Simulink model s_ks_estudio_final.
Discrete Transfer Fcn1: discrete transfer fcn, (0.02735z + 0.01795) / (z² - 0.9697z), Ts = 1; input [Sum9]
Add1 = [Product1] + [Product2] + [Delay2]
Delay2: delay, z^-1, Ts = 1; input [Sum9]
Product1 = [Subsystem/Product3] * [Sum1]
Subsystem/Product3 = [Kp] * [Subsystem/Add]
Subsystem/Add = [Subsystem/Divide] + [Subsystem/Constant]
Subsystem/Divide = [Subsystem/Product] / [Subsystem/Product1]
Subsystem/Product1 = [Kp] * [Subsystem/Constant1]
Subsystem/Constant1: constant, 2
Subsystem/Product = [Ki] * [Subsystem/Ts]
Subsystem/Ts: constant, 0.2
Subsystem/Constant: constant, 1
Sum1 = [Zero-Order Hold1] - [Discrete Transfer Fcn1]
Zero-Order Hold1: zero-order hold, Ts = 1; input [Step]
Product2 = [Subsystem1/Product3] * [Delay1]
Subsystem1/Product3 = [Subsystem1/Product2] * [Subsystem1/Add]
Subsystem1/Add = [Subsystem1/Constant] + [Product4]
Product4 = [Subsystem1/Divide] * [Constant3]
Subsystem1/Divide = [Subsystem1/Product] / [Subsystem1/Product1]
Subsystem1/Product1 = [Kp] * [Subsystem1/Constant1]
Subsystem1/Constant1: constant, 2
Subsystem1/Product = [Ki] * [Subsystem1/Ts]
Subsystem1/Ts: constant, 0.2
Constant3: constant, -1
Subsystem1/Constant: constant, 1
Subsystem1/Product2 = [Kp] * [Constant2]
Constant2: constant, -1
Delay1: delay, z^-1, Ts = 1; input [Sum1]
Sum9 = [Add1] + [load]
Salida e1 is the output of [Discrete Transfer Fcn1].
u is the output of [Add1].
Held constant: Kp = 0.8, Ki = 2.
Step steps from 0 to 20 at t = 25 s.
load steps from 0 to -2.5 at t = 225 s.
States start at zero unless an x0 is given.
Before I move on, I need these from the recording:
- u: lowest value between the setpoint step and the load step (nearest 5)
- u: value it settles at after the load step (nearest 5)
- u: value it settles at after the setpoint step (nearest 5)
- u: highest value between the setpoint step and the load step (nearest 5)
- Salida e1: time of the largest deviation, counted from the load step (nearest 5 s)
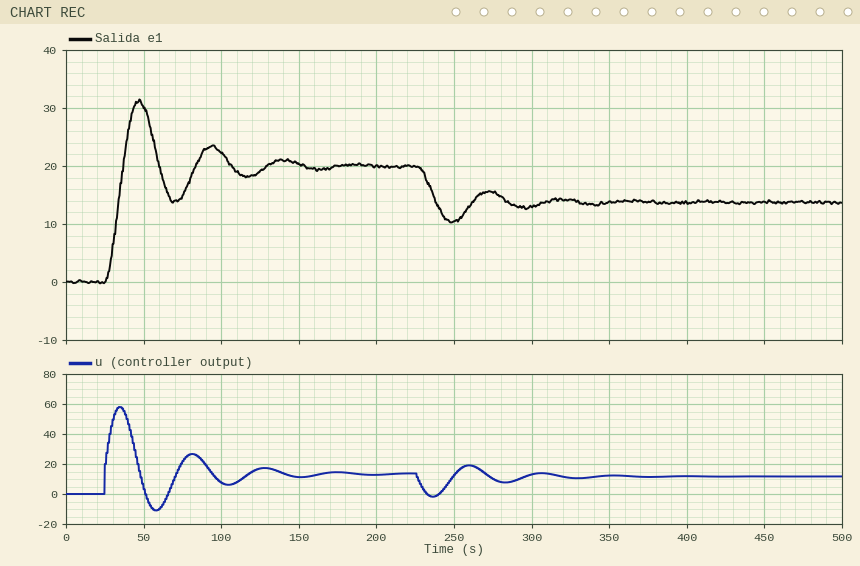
-10
10
15
60
25 s
